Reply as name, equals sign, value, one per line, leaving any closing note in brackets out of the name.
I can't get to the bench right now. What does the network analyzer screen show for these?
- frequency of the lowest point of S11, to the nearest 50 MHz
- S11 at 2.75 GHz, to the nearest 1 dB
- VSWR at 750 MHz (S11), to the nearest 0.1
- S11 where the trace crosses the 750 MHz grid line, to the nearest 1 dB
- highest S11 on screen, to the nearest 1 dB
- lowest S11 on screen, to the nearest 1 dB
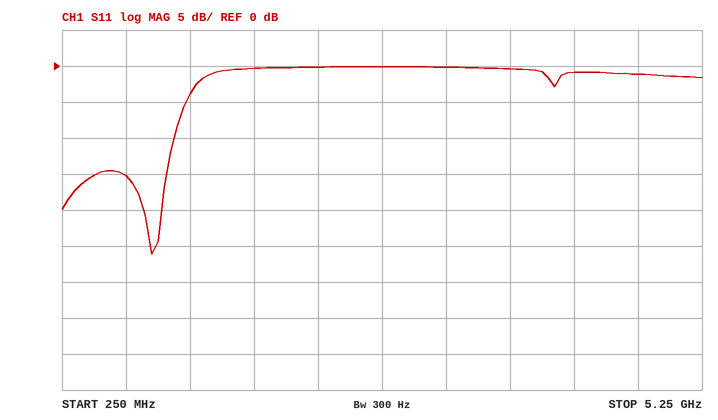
frequency of the lowest point of S11, to the nearest 50 MHz = 950 MHz
S11 at 2.75 GHz, to the nearest 1 dB = 0 dB
VSWR at 750 MHz (S11), to the nearest 0.1 = 1.4
S11 where the trace crosses the 750 MHz grid line, to the nearest 1 dB = -15 dB
highest S11 on screen, to the nearest 1 dB = 0 dB
lowest S11 on screen, to the nearest 1 dB = -26 dB
